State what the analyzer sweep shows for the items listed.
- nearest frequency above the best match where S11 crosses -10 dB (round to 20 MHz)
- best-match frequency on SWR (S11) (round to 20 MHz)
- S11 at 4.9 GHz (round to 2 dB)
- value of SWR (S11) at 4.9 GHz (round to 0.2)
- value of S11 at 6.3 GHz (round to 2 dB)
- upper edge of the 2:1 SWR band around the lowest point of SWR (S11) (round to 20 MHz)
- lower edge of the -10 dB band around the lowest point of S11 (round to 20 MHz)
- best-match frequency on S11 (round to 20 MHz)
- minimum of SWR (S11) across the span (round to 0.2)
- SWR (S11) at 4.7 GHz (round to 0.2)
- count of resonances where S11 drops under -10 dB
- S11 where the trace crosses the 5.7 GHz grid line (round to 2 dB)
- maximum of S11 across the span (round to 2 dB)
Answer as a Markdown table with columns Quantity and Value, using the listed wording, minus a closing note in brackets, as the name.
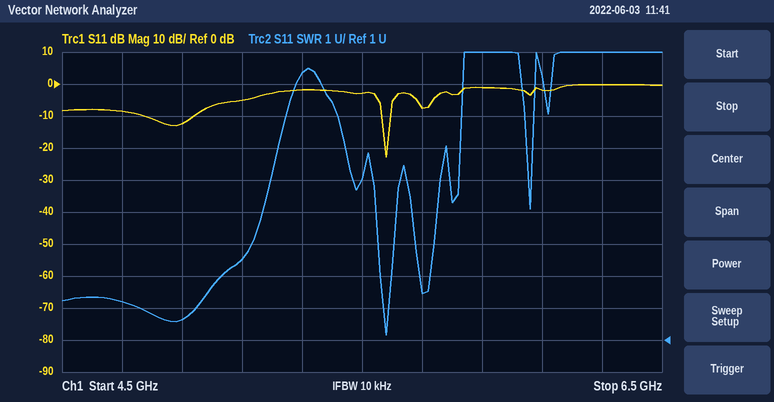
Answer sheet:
| Quantity | Value |
|---|---|
| nearest frequency above the best match where S11 crosses -10 dB | 5.60 GHz |
| best-match frequency on SWR (S11) | 5.58 GHz |
| S11 at 4.9 GHz | -12 dB |
| value of SWR (S11) at 4.9 GHz | 1.6 |
| value of S11 at 6.3 GHz | 0 dB |
| upper edge of the 2:1 SWR band around the lowest point of SWR (S11) | 5.58 GHz |
| lower edge of the -10 dB band around the lowest point of S11 | 5.56 GHz |
| best-match frequency on S11 | 5.58 GHz |
| minimum of SWR (S11) across the span | 1.2 |
| SWR (S11) at 4.7 GHz | 2.2 |
| count of resonances where S11 drops under -10 dB | 2 |
| S11 where the trace crosses the 5.7 GHz grid line | -8 dB |
| maximum of S11 across the span | 0 dB |
